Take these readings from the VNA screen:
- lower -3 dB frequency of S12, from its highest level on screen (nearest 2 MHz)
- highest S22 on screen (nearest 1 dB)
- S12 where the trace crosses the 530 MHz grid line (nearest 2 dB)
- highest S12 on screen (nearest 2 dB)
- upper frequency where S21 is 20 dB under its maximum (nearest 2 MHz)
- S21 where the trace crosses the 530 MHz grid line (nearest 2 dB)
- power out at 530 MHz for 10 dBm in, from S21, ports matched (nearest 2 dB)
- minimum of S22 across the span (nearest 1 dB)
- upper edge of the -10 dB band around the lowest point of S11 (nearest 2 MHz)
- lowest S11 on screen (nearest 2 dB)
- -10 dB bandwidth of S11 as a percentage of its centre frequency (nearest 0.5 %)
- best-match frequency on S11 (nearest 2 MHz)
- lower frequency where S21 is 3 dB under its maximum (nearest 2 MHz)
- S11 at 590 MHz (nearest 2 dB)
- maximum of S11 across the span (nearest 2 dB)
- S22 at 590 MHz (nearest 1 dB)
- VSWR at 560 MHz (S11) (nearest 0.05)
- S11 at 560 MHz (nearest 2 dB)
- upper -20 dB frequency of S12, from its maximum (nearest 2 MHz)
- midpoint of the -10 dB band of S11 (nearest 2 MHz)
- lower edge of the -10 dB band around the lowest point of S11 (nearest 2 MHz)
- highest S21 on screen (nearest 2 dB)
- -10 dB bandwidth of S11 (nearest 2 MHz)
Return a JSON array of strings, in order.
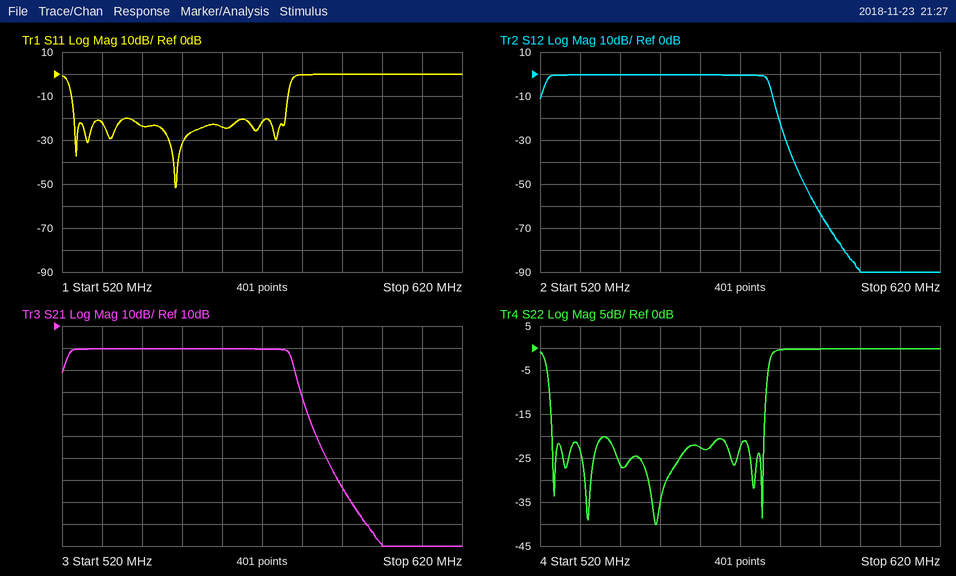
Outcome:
["522 MHz", "0 dB", "0 dB", "0 dB", "580 MHz", "0 dB", "10 dBm", "-40 dB", "576 MHz", "-52 dB", "10.0 %", "548 MHz", "522 MHz", "0 dB", "0 dB", "0 dB", "1.15", "-24 dB", "580 MHz", "550 MHz", "522 MHz", "0 dB", "54 MHz"]
